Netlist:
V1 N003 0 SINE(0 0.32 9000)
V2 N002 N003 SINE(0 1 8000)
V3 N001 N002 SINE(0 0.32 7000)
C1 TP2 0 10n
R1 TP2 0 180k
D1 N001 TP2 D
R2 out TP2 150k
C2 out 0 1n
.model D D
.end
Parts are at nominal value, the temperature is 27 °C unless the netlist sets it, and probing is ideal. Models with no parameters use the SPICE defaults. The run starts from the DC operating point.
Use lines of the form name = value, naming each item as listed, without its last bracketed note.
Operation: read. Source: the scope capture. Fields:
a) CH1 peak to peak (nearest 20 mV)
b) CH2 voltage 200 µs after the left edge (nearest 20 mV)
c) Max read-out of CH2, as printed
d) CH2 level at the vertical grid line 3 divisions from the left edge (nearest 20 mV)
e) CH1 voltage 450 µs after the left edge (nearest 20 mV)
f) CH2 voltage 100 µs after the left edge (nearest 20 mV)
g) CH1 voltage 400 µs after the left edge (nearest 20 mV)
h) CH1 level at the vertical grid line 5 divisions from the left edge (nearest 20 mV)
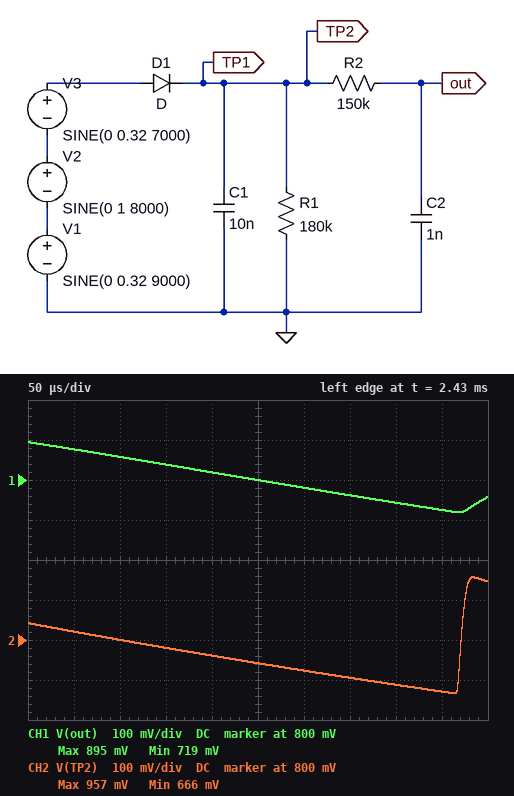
CH1 peak to peak = 180 mV
CH2 voltage 200 µs after the left edge = 760 mV
Max read-out of CH2, as printed = 957 mV
CH2 level at the vertical grid line 3 divisions from the left edge = 780 mV
CH1 voltage 450 µs after the left edge = 720 mV
CH2 voltage 100 µs after the left edge = 800 mV
CH1 voltage 400 µs after the left edge = 740 mV
CH1 level at the vertical grid line 5 divisions from the left edge = 800 mV
